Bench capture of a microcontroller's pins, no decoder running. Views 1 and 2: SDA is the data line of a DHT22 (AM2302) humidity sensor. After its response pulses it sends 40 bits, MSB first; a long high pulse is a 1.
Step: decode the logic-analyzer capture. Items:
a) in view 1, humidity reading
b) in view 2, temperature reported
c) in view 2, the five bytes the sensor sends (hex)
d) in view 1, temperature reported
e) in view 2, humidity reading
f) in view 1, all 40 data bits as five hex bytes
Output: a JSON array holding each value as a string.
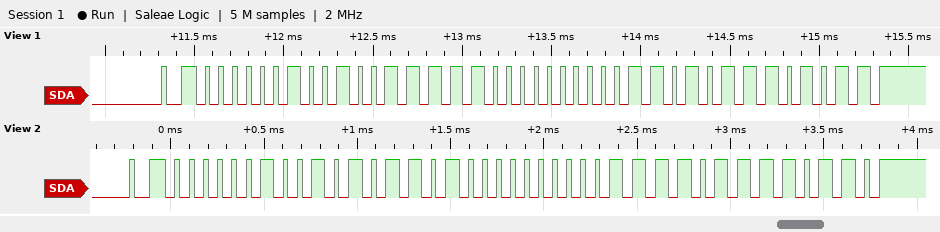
["59.1 %", "-3.0 °C", "02 56 80 1E F6", "-2.6 °C", "59.8 %", "02 4F 80 1A EB"]
